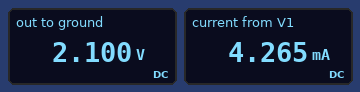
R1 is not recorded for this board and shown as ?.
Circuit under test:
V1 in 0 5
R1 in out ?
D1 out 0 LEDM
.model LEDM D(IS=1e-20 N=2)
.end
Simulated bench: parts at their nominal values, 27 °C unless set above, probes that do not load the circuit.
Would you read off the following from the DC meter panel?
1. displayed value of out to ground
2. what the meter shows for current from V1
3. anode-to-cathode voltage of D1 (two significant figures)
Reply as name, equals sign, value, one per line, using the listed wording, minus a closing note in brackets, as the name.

displayed value of out to ground = 2.100 V
what the meter shows for current from V1 = 4.265 mA
anode-to-cathode voltage of D1 = 2.1 V
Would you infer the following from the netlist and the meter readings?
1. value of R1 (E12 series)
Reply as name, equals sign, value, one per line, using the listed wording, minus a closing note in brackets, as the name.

value of R1 = 680 Ω
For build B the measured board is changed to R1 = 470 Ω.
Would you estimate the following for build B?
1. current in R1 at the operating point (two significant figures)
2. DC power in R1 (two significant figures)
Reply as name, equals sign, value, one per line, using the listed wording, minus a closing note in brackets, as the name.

current in R1 at the operating point = 6.1 mA
DC power in R1 = 18 mW
